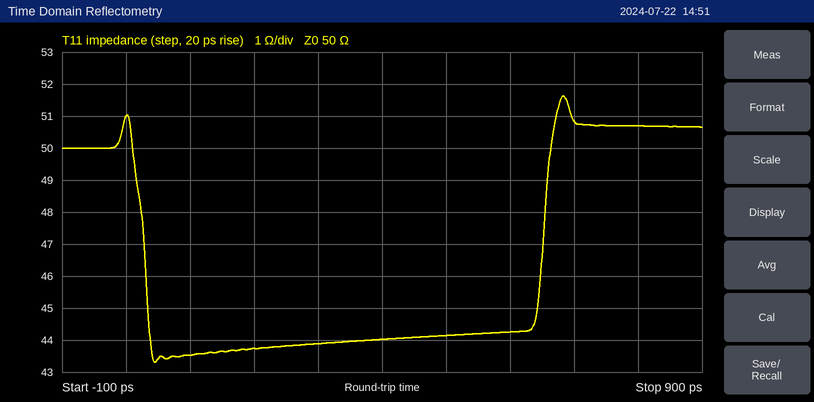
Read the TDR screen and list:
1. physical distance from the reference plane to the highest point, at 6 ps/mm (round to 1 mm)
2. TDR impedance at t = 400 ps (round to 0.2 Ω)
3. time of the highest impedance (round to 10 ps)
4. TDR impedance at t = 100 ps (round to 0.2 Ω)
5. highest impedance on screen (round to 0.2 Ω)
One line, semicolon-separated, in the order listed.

57 mm; 44.0 Ω; 680 ps; 43.6 Ω; 51.6 Ω
